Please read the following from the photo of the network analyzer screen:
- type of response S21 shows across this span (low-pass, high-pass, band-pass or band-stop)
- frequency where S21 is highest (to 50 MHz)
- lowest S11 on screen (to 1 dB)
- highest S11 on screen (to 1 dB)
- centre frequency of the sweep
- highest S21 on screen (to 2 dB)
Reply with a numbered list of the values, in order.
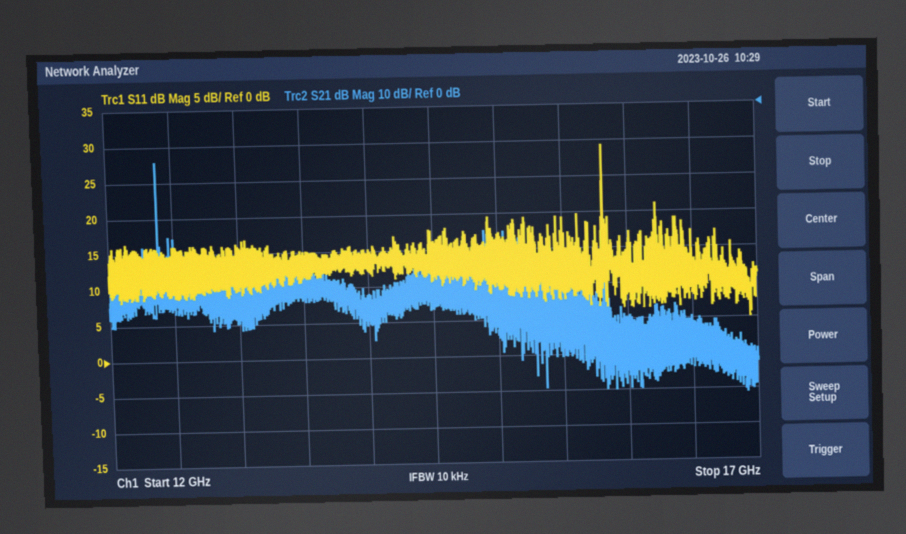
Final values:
1. band-pass
2. 12.40 GHz
3. 5 dB
4. 29 dB
5. 14.5 GHz
6. -14 dB
